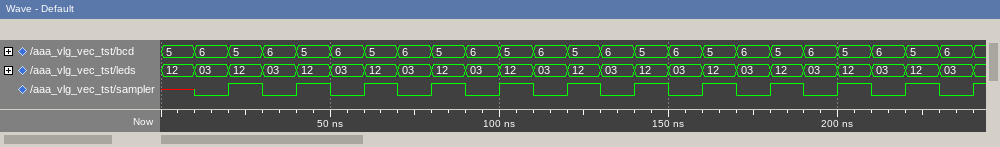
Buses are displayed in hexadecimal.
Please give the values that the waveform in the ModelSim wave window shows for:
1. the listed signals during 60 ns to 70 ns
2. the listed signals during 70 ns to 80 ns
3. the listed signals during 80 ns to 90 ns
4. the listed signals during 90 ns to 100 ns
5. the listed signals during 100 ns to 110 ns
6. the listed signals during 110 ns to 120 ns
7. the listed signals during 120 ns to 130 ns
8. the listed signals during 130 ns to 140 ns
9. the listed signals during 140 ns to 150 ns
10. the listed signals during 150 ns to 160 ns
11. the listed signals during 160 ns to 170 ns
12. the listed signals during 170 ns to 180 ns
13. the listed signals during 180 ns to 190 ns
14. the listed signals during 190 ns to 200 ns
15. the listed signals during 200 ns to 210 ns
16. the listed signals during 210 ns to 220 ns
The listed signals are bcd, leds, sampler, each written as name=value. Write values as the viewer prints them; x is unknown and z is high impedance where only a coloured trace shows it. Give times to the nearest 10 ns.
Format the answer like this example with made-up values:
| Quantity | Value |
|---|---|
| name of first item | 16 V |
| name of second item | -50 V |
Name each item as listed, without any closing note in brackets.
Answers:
| Quantity | Value |
|---|---|
| the listed signals during 60 ns to 70 ns | bcd=5, leds=12, sampler=1 |
| the listed signals during 70 ns to 80 ns | bcd=6, leds=03, sampler=0 |
| the listed signals during 80 ns to 90 ns | bcd=5, leds=12, sampler=1 |
| the listed signals during 90 ns to 100 ns | bcd=6, leds=03, sampler=0 |
| the listed signals during 100 ns to 110 ns | bcd=5, leds=12, sampler=1 |
| the listed signals during 110 ns to 120 ns | bcd=6, leds=03, sampler=0 |
| the listed signals during 120 ns to 130 ns | bcd=5, leds=12, sampler=1 |
| the listed signals during 130 ns to 140 ns | bcd=6, leds=03, sampler=0 |
| the listed signals during 140 ns to 150 ns | bcd=5, leds=12, sampler=1 |
| the listed signals during 150 ns to 160 ns | bcd=6, leds=03, sampler=0 |
| the listed signals during 160 ns to 170 ns | bcd=5, leds=12, sampler=1 |
| the listed signals during 170 ns to 180 ns | bcd=6, leds=03, sampler=0 |
| the listed signals during 180 ns to 190 ns | bcd=5, leds=12, sampler=1 |
| the listed signals during 190 ns to 200 ns | bcd=6, leds=03, sampler=0 |
| the listed signals during 200 ns to 210 ns | bcd=5, leds=12, sampler=1 |
| the listed signals during 210 ns to 220 ns | bcd=6, leds=03, sampler=0 |
